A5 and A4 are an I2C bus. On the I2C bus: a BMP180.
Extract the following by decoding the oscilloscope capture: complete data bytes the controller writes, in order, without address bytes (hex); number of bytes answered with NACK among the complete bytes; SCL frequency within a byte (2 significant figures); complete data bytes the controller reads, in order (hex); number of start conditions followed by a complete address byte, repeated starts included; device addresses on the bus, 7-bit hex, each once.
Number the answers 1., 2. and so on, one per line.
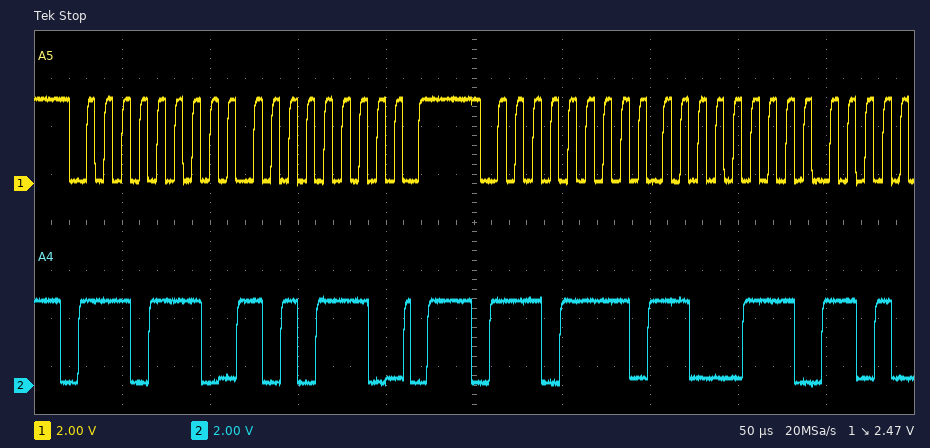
1. AE
2. 0
3. 100 kHz
4. C7
5. 2
6. 0x77
